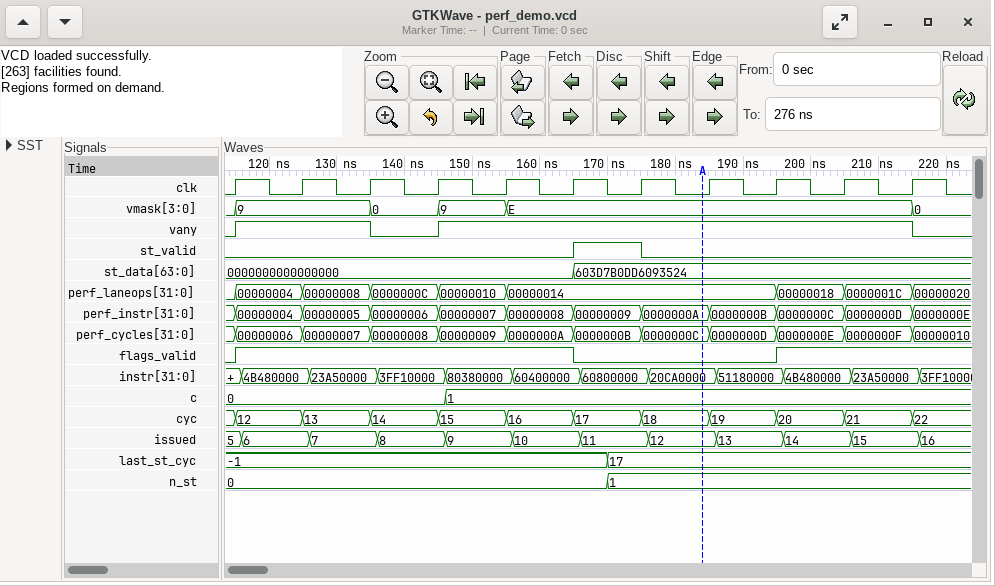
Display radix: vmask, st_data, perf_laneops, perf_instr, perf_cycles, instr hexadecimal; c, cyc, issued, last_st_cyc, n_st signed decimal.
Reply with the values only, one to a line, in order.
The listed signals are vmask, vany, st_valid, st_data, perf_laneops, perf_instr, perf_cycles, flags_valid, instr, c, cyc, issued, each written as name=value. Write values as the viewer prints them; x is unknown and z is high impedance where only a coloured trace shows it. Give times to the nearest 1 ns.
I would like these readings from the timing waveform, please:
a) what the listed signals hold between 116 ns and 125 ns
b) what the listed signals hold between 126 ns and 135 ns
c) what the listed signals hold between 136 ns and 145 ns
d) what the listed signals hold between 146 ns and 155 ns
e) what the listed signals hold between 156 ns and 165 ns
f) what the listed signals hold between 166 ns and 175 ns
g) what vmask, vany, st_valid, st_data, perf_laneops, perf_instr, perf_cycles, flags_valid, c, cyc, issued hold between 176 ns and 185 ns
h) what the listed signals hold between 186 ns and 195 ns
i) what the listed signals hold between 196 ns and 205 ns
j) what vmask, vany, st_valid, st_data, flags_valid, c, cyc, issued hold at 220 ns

vmask=9, vany=1, st_valid=0, st_data=0000000000000000, perf_laneops=00000004, perf_instr=00000004, perf_cycles=00000006, flags_valid=1, instr=4B480000, c=0, cyc=12, issued=6
vmask=9, vany=1, st_valid=0, st_data=0000000000000000, perf_laneops=00000008, perf_instr=00000005, perf_cycles=00000007, flags_valid=1, instr=23A50000, c=0, cyc=13, issued=7
vmask=0, vany=0, st_valid=0, st_data=0000000000000000, perf_laneops=0000000C, perf_instr=00000006, perf_cycles=00000008, flags_valid=1, instr=3FF10000, c=0, cyc=14, issued=8
vmask=9, vany=1, st_valid=0, st_data=0000000000000000, perf_laneops=00000010, perf_instr=00000007, perf_cycles=00000009, flags_valid=1, instr=80380000, c=1, cyc=15, issued=9
vmask=E, vany=1, st_valid=0, st_data=0000000000000000, perf_laneops=00000014, perf_instr=00000008, perf_cycles=0000000A, flags_valid=1, instr=60400000, c=1, cyc=16, issued=10
vmask=E, vany=1, st_valid=1, st_data=603D7B0DD6093524, perf_laneops=00000014, perf_instr=00000009, perf_cycles=0000000B, flags_valid=0, instr=60800000, c=1, cyc=17, issued=11
vmask=E, vany=1, st_valid=0, st_data=603D7B0DD6093524, perf_laneops=00000014, perf_instr=0000000A, perf_cycles=0000000C, flags_valid=0, c=1, cyc=18, issued=12
vmask=E, vany=1, st_valid=0, st_data=603D7B0DD6093524, perf_laneops=00000014, perf_instr=0000000B, perf_cycles=0000000D, flags_valid=0, instr=51180000, c=1, cyc=19, issued=13
vmask=E, vany=1, st_valid=0, st_data=603D7B0DD6093524, perf_laneops=00000018, perf_instr=0000000C, perf_cycles=0000000E, flags_valid=1, instr=4B480000, c=1, cyc=20, issued=14
vmask=0, vany=0, st_valid=0, st_data=603D7B0DD6093524, flags_valid=1, c=1, cyc=22, issued=16
